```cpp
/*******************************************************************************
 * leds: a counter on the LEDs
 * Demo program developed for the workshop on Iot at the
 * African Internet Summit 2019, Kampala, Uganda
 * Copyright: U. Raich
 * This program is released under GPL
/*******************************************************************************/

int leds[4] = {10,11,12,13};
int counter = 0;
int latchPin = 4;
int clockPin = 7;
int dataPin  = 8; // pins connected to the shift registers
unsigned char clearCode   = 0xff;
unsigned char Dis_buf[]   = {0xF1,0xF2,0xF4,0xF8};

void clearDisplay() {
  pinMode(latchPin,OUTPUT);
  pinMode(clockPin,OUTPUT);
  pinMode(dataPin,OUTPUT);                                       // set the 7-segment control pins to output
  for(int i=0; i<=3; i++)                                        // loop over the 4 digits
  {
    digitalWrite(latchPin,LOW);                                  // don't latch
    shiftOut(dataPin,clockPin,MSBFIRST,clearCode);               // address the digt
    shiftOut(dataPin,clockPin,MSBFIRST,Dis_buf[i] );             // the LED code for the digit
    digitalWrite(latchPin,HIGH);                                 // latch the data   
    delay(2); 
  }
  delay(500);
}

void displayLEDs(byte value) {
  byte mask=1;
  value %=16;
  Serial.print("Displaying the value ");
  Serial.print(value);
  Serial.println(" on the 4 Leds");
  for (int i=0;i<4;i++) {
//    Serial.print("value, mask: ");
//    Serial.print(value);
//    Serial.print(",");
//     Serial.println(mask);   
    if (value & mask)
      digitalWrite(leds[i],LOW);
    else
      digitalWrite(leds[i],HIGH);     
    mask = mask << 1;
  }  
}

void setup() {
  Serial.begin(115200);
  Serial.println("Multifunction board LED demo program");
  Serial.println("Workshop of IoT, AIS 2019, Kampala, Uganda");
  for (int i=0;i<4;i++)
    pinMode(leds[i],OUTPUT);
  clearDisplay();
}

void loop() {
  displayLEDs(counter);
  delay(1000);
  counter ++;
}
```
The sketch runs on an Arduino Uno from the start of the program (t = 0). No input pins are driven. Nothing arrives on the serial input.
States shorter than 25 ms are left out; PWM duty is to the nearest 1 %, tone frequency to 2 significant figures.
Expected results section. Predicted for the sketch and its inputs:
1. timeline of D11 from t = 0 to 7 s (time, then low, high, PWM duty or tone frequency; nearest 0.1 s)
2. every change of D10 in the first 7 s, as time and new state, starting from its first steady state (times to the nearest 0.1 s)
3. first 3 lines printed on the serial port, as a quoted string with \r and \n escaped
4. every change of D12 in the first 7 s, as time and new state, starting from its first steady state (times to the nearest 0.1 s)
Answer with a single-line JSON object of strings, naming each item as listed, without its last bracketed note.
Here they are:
{"timeline of D11 from t = 0 to 7 s": "0 s low; 0.5 s high; 2.5 s low; 4.5 s high; 6.5 s low", "every change of D10 in the first 7 s, as time and new state, starting from its first steady state": "0 s low; 0.5 s high; 1.5 s low; 2.5 s high; 3.5 s low; 4.5 s high; 5.5 s low; 6.5 s high", "first 3 lines printed on the serial port, as a quoted string with \\r and \\n escaped": "\"Multifunction board LED demo program\\r\\nWorkshop of IoT, AIS 2019, Kampala, Uganda\\r\\nDisplaying the value 0 on the 4 Leds\\r\\n\"", "every change of D12 in the first 7 s, as time and new state, starting from its first steady state": "0 s low; 0.5 s high; 4.5 s low"}
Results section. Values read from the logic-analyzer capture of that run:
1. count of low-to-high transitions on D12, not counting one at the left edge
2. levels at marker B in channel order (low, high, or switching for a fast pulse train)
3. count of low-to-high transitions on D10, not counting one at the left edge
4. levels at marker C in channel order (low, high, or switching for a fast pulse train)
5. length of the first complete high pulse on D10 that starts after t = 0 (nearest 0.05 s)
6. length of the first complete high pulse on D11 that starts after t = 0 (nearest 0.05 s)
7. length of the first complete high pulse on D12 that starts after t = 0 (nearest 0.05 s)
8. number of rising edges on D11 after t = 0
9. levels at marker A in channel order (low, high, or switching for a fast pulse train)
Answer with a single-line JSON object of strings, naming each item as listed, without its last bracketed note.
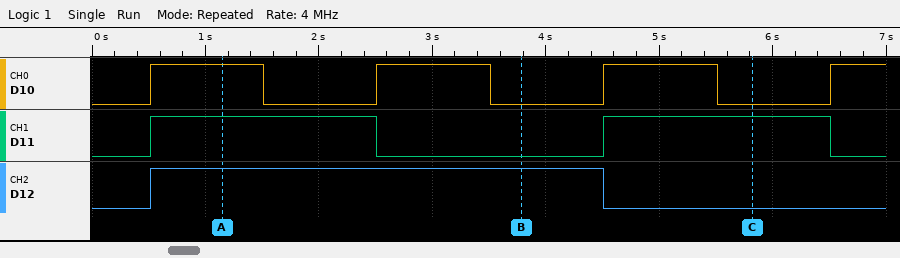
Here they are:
{"count of low-to-high transitions on D12, not counting one at the left edge": "1", "levels at marker B in channel order": "D10 low, D11 low, D12 high", "count of low-to-high transitions on D10, not counting one at the left edge": "4", "levels at marker C in channel order": "D10 low, D11 high, D12 low", "length of the first complete high pulse on D10 that starts after t = 0": "1.00 s", "length of the first complete high pulse on D11 that starts after t = 0": "2.00 s", "length of the first complete high pulse on D12 that starts after t = 0": "4.00 s", "number of rising edges on D11 after t = 0": "2", "levels at marker A in channel order": "D10 high, D11 high, D12 high"}
